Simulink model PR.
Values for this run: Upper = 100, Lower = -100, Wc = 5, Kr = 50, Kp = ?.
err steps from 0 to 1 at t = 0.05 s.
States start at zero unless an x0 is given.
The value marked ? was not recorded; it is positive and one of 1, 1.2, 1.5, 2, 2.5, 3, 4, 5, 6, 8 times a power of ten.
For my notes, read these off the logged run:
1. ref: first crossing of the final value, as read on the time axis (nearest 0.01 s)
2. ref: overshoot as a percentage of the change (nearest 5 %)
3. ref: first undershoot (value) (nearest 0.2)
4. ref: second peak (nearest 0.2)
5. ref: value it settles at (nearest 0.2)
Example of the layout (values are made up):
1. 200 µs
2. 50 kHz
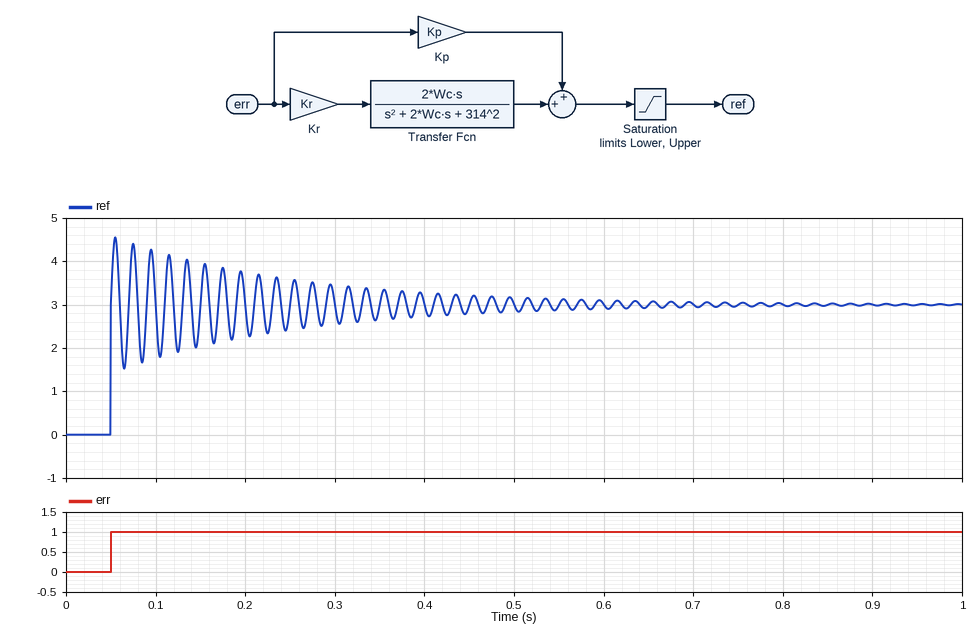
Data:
1. 0.05 s
2. 50 %
3. 1.6
4. 4.4
5. 3.0
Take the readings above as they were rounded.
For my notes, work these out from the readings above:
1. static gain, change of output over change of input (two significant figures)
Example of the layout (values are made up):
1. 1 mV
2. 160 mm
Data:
1. 3.0
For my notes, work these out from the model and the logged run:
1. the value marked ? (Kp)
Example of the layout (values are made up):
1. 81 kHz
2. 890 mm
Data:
1. 3
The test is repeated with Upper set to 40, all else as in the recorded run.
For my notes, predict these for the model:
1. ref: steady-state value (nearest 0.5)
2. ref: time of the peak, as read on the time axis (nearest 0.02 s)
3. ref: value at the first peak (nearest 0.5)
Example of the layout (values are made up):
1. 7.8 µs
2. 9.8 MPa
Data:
1. 3.0
2. 0.06 s
3. 4.5
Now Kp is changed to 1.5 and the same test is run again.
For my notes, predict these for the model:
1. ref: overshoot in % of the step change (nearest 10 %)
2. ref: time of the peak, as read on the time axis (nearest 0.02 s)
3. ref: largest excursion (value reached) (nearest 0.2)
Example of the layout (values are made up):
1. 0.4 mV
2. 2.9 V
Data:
1. 100 %
2. 0.06 s
3. 3.0
